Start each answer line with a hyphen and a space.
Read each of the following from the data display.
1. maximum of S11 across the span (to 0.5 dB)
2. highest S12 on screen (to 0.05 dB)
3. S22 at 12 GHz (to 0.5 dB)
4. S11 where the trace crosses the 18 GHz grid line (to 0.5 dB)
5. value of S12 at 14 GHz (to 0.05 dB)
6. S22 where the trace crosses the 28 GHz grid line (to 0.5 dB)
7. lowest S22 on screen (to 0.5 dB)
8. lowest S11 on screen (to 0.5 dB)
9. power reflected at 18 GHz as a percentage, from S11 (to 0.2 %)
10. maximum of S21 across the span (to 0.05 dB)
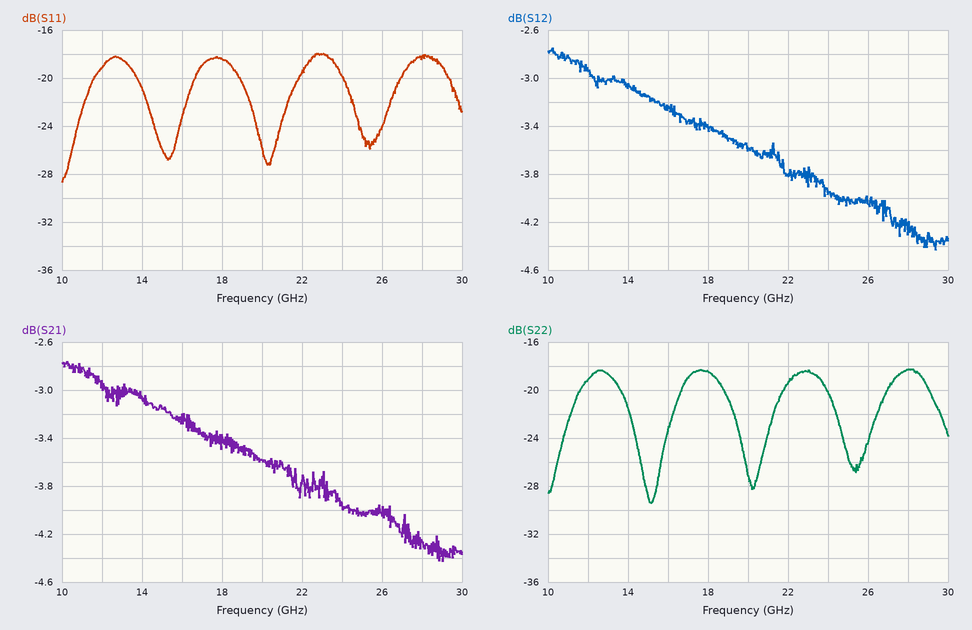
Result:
- -18.0 dB
- -2.75 dB
- -19.0 dB
- -18.5 dB
- -3.05 dB
- -18.5 dB
- -29.5 dB
- -28.5 dB
- 1.4 %
- -2.75 dB
